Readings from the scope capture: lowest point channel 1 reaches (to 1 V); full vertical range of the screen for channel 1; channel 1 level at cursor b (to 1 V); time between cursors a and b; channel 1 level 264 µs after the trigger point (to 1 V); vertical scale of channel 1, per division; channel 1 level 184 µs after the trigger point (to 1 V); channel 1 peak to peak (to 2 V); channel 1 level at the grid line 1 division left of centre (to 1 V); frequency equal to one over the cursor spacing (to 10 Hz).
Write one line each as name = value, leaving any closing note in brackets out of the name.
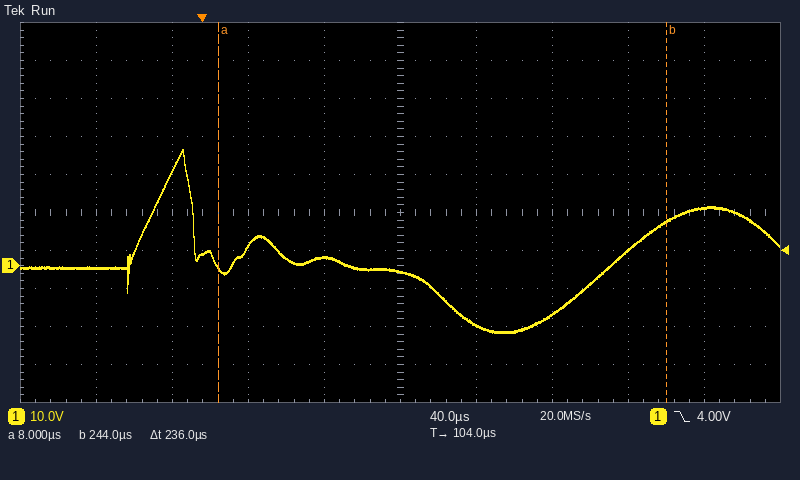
lowest point channel 1 reaches = -18 V
full vertical range of the screen for channel 1 = 100 V
channel 1 level at cursor b = 12 V
time between cursors a and b = 236 µs
channel 1 level 264 µs after the trigger point = 15 V
vertical scale of channel 1, per division = 10 V
channel 1 level 184 µs after the trigger point = -13 V
channel 1 peak to peak = 48 V
channel 1 level at the grid line 1 division left of centre = 2 V
frequency equal to one over the cursor spacing = 4.24 kHz
